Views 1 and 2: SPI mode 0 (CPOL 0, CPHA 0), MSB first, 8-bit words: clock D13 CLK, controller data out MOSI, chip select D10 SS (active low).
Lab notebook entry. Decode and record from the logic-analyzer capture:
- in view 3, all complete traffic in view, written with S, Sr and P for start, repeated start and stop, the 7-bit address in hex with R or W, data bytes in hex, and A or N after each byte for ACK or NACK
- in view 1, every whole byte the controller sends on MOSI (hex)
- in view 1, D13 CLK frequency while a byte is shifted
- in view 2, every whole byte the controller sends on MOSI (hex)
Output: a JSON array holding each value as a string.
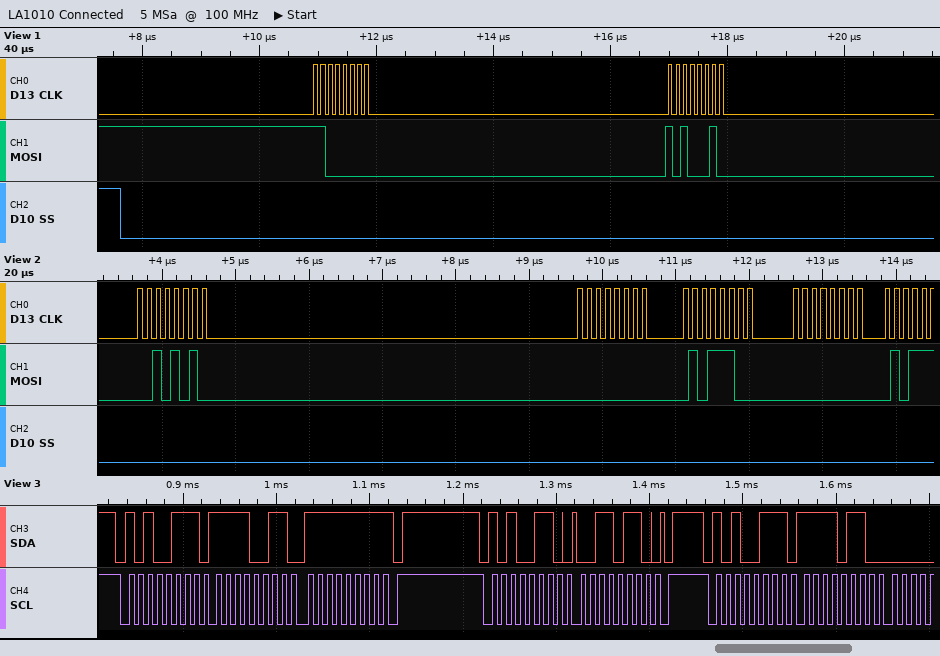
["S 53R A F3 A FF N P S 53W A 36 A P S 53R A F6 A", "C0 A2", "8 MHz", "0x2A 0x00 0x5C 0x00"]
